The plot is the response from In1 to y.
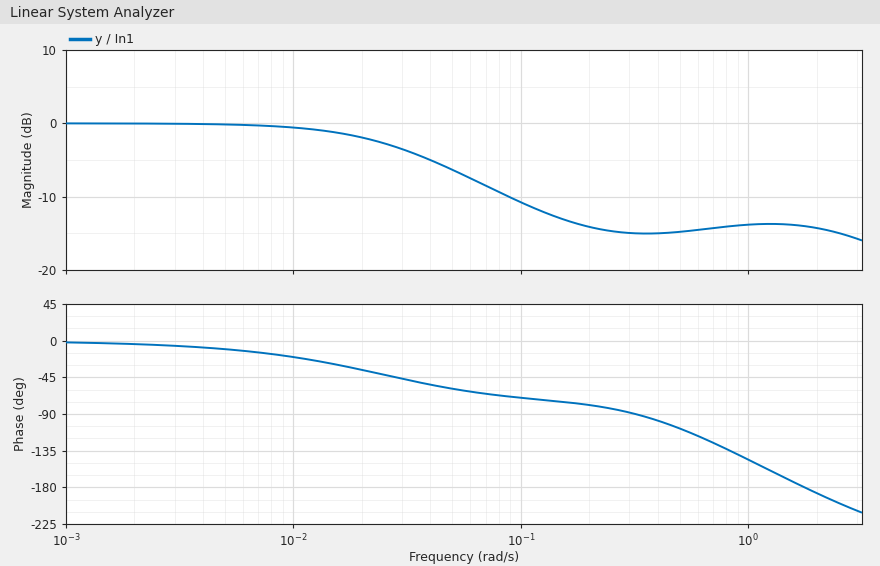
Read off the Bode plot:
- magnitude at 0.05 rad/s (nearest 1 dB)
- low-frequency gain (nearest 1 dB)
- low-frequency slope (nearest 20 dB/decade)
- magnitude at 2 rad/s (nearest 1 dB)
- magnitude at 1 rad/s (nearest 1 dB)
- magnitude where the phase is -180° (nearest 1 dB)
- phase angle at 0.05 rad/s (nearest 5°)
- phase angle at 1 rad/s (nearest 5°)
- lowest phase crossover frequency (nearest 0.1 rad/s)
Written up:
-6 dB
0 dB
0 dB/decade
-14 dB
-14 dB
-14 dB
-60°
-145°
1.8 rad/s
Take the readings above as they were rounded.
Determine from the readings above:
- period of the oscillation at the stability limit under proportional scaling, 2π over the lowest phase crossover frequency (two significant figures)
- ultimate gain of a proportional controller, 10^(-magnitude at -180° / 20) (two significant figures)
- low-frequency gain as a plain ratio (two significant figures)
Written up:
3.5 s
5.0
1.0
